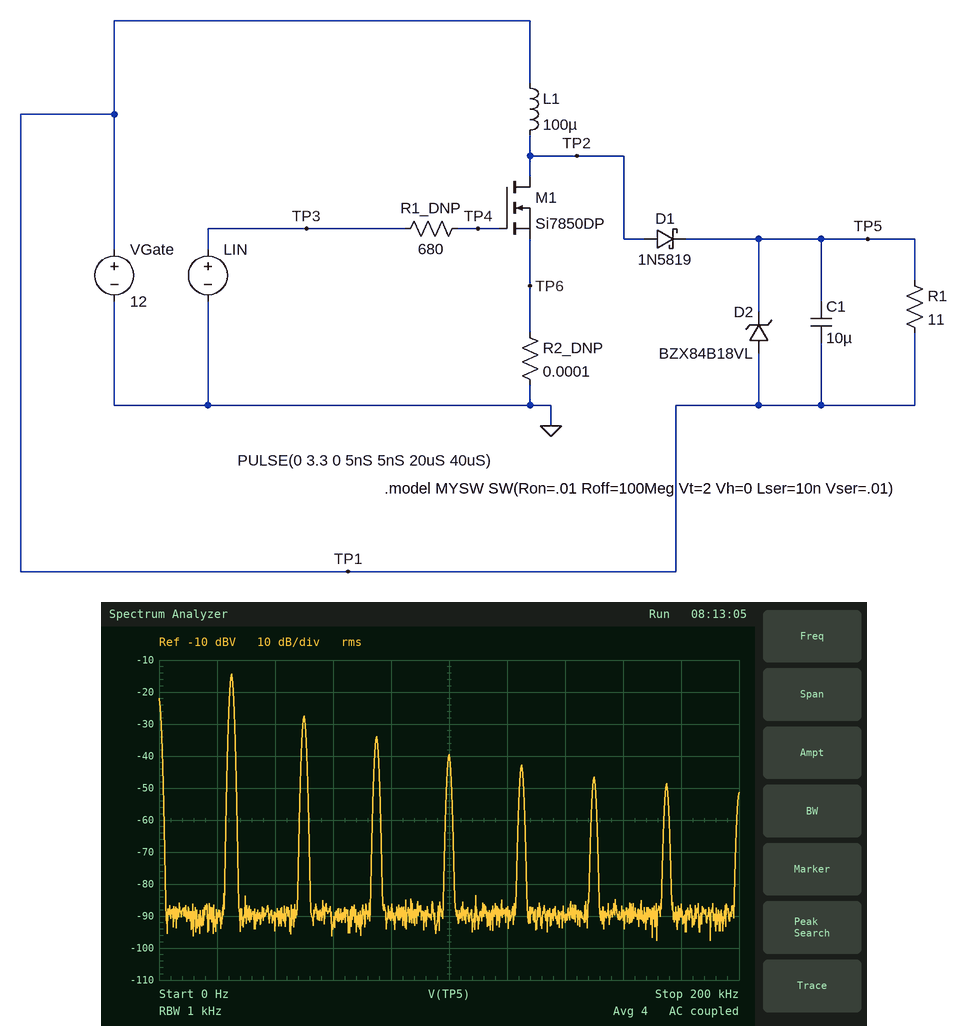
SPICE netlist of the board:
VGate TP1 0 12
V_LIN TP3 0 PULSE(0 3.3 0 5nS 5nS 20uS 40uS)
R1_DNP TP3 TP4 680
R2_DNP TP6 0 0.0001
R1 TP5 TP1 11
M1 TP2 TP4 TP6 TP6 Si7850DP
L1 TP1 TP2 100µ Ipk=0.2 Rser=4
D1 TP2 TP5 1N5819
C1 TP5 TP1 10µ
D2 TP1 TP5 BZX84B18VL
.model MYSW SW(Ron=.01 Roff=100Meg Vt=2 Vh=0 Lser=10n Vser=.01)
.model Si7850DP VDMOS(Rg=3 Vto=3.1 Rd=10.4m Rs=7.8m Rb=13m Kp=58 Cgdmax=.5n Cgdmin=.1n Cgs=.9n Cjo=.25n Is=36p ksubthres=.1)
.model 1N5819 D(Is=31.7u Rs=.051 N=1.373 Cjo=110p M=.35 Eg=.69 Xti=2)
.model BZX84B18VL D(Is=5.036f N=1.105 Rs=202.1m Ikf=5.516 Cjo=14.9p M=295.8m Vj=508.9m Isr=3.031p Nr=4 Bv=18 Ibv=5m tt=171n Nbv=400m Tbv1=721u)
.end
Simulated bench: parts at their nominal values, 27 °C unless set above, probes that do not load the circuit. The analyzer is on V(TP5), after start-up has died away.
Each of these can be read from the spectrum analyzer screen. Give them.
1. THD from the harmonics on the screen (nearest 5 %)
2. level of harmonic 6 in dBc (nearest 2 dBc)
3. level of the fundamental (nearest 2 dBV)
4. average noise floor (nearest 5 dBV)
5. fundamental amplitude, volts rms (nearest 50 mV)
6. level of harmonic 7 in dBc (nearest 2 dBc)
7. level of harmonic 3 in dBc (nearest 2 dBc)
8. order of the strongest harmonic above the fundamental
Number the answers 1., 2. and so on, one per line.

1. 25 %
2. -32 dBc
3. -14 dBV
4. -90 dBV
5. 200 mV
6. -34 dBc
7. -20 dBc
8. 2
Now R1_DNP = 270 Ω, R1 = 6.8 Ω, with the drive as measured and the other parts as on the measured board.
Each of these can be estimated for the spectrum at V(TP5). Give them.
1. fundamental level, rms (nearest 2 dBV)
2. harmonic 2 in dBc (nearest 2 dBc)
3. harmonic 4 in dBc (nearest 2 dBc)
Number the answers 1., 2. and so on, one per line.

1. -12 dBV
2. -14 dBc
3. -26 dBc
